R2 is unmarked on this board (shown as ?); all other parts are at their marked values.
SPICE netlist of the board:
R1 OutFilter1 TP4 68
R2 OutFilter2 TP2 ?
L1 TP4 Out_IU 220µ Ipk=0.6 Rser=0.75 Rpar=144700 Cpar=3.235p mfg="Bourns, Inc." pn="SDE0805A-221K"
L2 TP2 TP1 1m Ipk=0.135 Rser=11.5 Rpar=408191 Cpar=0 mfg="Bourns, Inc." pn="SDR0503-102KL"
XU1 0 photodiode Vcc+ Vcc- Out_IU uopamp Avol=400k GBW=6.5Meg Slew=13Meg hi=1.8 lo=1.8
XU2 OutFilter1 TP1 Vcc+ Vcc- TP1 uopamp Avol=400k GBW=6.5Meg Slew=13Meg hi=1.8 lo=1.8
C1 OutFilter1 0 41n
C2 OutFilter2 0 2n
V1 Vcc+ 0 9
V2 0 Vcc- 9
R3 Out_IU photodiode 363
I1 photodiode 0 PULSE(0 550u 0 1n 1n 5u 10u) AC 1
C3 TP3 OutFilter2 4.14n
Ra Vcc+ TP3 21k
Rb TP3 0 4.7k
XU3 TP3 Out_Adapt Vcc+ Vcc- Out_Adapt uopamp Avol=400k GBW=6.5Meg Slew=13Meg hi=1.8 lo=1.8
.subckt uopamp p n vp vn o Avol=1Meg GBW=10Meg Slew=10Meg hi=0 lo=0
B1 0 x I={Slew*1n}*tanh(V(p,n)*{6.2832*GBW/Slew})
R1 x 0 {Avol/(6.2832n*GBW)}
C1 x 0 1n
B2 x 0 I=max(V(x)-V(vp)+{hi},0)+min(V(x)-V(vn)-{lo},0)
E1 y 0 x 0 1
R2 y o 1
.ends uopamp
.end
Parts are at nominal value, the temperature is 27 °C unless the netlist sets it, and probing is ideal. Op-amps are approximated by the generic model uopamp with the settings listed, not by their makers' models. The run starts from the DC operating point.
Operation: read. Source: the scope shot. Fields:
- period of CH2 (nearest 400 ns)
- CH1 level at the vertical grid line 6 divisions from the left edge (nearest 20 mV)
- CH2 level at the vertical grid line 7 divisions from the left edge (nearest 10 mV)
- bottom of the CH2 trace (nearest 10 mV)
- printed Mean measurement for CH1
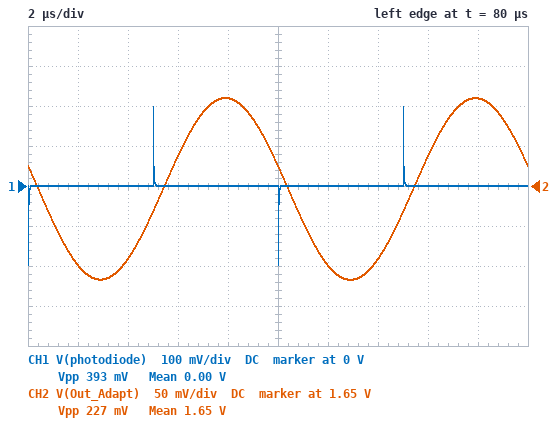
10.0 µs
0 V
1.56 V
1.53 V
0.00 V
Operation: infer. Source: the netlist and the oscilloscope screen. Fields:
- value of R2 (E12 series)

82 Ω
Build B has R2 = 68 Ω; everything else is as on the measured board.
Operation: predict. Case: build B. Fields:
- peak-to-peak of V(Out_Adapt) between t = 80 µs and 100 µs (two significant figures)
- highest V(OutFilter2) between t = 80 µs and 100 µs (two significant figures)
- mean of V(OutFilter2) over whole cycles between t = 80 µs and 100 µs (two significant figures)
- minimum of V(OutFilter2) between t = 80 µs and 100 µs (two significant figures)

240 mV
220 mV
100 mV
-20 mV
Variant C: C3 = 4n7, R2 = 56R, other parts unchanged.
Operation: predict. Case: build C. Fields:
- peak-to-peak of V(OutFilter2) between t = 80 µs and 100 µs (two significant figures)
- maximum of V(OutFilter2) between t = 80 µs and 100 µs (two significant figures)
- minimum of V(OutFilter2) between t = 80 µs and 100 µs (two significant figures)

250 mV
220 mV
-24 mV
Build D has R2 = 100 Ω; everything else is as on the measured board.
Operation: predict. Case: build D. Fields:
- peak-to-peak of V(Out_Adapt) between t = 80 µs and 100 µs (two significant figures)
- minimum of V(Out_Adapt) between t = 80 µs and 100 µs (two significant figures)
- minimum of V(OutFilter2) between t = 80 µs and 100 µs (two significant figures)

210 mV
1.5 V
-7.8 mV
